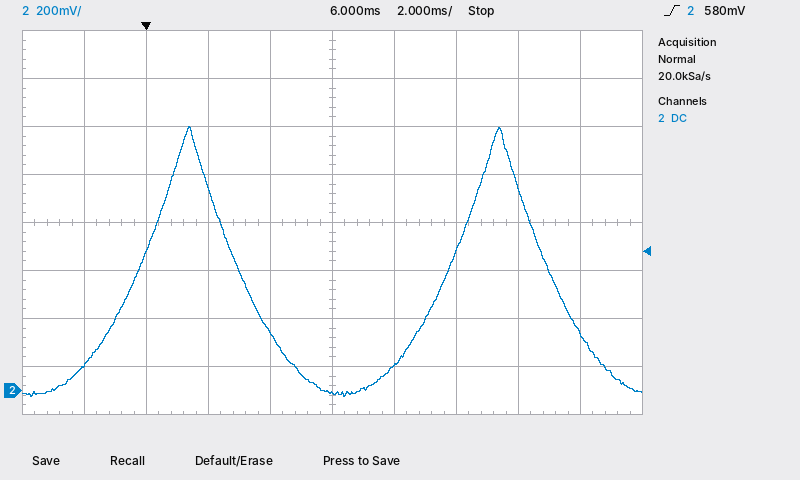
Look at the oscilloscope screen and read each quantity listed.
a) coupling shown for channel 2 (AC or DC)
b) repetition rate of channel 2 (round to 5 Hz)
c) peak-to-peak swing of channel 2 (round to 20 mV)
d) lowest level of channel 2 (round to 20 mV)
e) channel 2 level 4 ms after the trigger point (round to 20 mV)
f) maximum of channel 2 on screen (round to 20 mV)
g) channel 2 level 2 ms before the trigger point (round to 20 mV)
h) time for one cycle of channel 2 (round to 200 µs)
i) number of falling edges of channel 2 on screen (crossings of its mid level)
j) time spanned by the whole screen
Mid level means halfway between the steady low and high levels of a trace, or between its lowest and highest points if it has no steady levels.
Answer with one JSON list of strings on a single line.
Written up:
["DC", "100 Hz", "1.12 V", "-20 mV", "240 mV", "1.10 V", "100 mV", "10.0 ms", "2", "20 ms"]
